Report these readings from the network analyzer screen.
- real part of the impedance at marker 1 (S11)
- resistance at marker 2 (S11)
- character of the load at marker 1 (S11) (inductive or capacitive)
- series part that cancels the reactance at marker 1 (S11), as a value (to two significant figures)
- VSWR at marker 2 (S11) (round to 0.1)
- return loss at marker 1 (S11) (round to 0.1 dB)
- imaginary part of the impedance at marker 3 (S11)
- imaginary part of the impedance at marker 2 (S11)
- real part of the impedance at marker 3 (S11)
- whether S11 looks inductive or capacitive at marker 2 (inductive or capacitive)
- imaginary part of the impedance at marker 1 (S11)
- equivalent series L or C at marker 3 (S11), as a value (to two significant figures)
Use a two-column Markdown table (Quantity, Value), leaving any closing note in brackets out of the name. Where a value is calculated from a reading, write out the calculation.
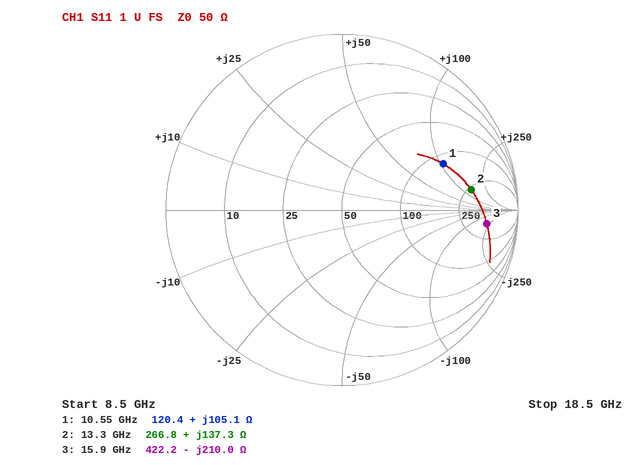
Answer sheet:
| Quantity | Value |
|---|---|
| real part of the impedance at marker 1 | 120.4 Ω |
| resistance at marker 2 | 266.8 Ω |
| character of the load at marker 1 (S11) | inductive |
| series part that cancels the reactance at marker 1 (S11), as a value | C = 1/(2π × 10.55 GHz × 105.1 Ω) ≈ 144 fF, so 140 fF to two significant figures |
| VSWR at marker 2 (S11) | 6.8 |
| return loss at marker 1 (S11) | 4.0 dB |
| imaginary part of the impedance at marker 3 | -210.0 Ω |
| imaginary part of the impedance at marker 2 | +137.3 Ω |
| real part of the impedance at marker 3 | 422.2 Ω |
| whether S11 looks inductive or capacitive at marker 2 | inductive |
| imaginary part of the impedance at marker 1 | +105.1 Ω |
| equivalent series L or C at marker 3 (S11), as a value | C = 1/(2π × 15.9 GHz × 210 Ω) ≈ 48 fF |
